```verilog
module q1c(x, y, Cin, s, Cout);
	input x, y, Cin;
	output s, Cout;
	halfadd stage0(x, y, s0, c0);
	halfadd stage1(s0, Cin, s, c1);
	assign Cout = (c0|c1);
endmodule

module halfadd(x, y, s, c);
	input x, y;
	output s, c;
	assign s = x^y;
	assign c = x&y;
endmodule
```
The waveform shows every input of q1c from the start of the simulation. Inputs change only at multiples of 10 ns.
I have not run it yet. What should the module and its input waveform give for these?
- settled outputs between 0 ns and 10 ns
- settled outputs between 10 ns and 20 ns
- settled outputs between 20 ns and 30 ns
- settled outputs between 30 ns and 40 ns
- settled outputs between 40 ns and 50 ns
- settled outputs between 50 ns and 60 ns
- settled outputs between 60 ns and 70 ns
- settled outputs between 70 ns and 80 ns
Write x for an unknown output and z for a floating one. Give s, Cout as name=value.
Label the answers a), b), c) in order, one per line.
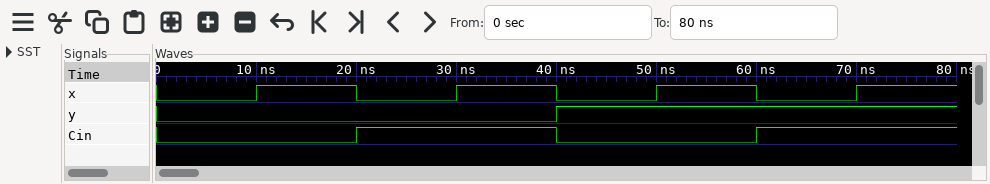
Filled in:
a) s=0, Cout=0
b) s=1, Cout=0
c) s=1, Cout=0
d) s=0, Cout=1
e) s=1, Cout=0
f) s=0, Cout=1
g) s=0, Cout=1
h) s=1, Cout=1
